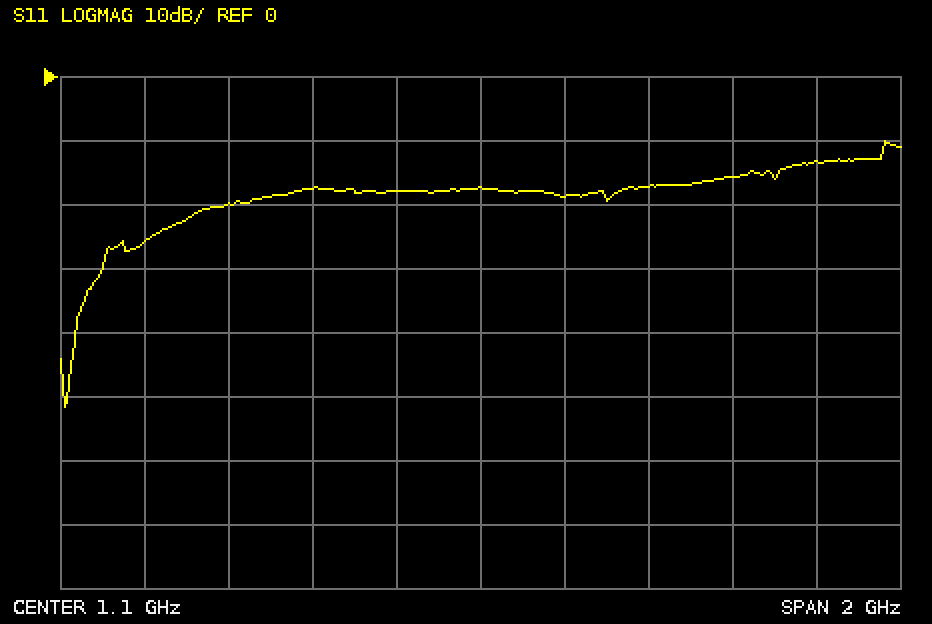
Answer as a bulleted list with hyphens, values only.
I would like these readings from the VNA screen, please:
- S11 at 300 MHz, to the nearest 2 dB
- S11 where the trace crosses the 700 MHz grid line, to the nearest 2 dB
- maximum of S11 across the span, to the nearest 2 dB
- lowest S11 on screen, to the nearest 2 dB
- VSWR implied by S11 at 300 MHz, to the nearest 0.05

- -26 dB
- -18 dB
- -10 dB
- -52 dB
- 1.10
